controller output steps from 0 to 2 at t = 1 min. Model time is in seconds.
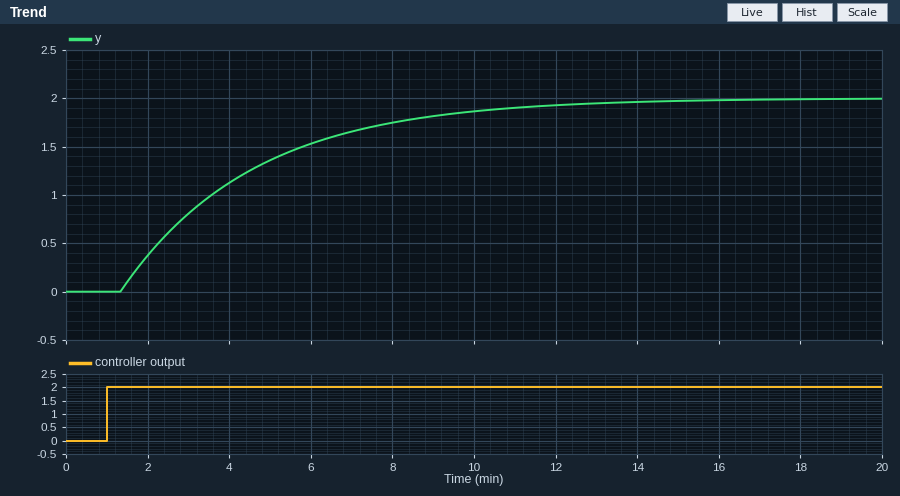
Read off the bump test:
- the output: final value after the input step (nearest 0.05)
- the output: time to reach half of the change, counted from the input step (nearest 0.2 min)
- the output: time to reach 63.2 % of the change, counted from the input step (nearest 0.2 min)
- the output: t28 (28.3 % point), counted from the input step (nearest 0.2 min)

2.00
2.6 min
3.6 min
1.4 min
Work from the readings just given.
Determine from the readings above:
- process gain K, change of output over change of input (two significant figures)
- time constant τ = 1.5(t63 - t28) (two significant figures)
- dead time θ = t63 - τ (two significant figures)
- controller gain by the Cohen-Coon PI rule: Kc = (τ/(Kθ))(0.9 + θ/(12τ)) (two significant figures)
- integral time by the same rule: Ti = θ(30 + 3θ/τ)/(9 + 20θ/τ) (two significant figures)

1.0
3.3 min
0.30 min
10.0
0.84 min
